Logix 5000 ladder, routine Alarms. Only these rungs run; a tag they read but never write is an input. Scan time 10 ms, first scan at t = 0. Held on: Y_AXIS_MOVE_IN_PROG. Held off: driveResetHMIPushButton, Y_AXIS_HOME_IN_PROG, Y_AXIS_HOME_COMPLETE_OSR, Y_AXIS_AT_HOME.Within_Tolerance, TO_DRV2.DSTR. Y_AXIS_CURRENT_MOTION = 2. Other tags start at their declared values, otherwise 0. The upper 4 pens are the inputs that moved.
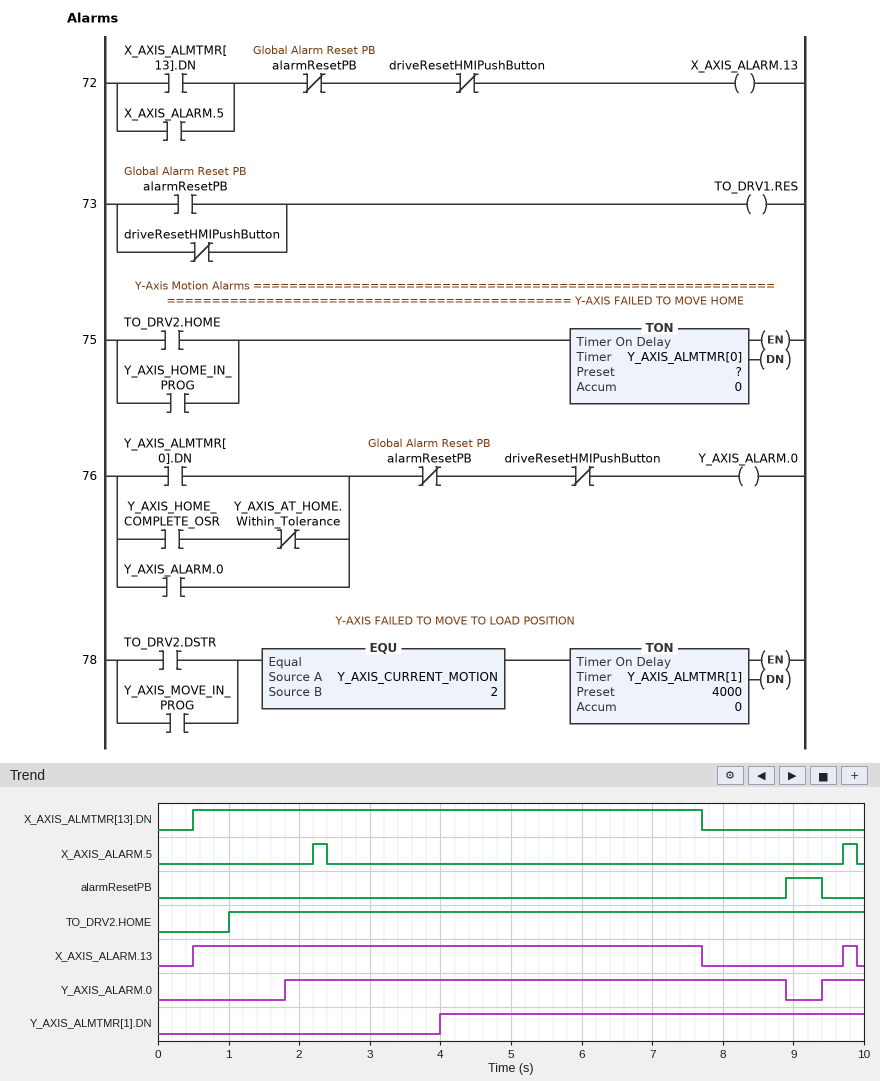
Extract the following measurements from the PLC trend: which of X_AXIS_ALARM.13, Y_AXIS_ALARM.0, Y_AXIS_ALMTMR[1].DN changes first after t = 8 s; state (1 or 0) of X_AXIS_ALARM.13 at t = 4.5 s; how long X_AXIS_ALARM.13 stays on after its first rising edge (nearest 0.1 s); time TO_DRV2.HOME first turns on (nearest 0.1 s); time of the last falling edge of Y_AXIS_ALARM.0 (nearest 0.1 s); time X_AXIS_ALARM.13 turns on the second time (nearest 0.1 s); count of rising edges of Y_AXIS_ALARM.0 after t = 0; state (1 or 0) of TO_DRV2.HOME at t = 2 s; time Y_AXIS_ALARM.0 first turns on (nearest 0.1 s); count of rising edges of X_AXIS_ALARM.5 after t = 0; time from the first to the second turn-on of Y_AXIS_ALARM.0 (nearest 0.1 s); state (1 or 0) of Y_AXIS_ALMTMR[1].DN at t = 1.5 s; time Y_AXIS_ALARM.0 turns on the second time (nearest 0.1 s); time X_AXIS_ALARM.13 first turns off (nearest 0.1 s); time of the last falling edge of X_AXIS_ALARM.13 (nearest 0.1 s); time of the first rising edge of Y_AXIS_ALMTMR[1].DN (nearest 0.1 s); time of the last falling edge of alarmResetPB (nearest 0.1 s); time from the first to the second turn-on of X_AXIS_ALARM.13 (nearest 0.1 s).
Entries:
Y_AXIS_ALARM.0
1
7.2 s
1.0 s
8.9 s
9.7 s
2
1
1.8 s
2
7.6 s
0
9.4 s
7.7 s
9.9 s
4.0 s
9.4 s
9.2 s
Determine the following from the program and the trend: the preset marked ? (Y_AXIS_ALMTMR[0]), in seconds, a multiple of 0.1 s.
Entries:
0.8 s
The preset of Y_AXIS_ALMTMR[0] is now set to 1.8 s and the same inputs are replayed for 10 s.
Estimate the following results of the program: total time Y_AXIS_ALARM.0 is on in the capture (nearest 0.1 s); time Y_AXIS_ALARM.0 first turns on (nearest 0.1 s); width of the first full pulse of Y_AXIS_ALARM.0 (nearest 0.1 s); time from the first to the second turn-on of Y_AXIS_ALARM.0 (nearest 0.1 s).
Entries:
6.7 s
2.8 s
6.1 s
6.6 s
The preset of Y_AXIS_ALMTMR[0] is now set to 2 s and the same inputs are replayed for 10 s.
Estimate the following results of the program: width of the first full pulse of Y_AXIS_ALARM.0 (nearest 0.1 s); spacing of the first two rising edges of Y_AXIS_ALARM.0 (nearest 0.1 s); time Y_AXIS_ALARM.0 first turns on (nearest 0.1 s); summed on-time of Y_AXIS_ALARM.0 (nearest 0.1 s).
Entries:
5.9 s
6.4 s
3.0 s
6.5 s
